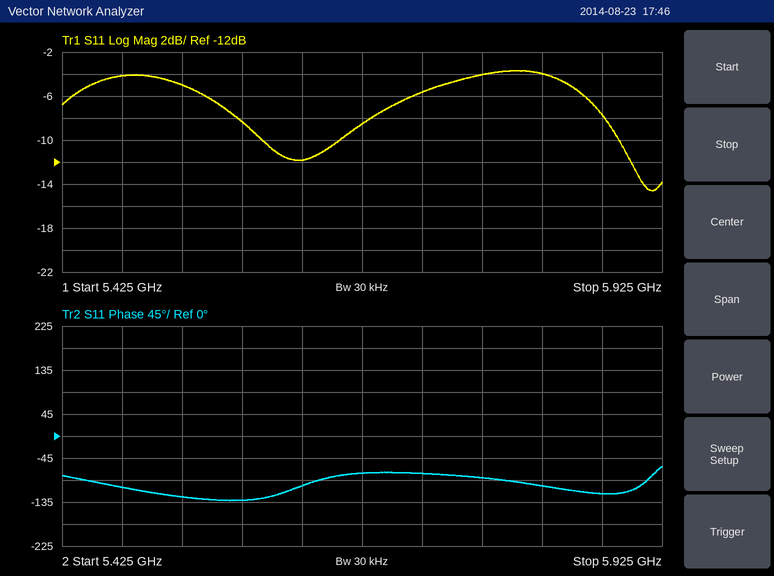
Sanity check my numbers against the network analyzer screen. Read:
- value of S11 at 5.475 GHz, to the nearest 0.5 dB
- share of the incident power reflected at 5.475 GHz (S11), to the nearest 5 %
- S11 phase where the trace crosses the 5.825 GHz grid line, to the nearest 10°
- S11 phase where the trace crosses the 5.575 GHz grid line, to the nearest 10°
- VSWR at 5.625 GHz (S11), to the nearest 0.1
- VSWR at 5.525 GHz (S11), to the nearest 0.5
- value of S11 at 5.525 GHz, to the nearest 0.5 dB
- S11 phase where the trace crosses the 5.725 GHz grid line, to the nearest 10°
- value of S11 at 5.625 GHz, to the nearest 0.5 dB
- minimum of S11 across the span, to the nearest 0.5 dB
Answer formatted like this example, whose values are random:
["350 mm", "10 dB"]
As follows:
["-4.0 dB", "40 %", "-100°", "-130°", "1.7", "3.5", "-5.0 dB", "-80°", "-12.0 dB", "-14.5 dB"]
